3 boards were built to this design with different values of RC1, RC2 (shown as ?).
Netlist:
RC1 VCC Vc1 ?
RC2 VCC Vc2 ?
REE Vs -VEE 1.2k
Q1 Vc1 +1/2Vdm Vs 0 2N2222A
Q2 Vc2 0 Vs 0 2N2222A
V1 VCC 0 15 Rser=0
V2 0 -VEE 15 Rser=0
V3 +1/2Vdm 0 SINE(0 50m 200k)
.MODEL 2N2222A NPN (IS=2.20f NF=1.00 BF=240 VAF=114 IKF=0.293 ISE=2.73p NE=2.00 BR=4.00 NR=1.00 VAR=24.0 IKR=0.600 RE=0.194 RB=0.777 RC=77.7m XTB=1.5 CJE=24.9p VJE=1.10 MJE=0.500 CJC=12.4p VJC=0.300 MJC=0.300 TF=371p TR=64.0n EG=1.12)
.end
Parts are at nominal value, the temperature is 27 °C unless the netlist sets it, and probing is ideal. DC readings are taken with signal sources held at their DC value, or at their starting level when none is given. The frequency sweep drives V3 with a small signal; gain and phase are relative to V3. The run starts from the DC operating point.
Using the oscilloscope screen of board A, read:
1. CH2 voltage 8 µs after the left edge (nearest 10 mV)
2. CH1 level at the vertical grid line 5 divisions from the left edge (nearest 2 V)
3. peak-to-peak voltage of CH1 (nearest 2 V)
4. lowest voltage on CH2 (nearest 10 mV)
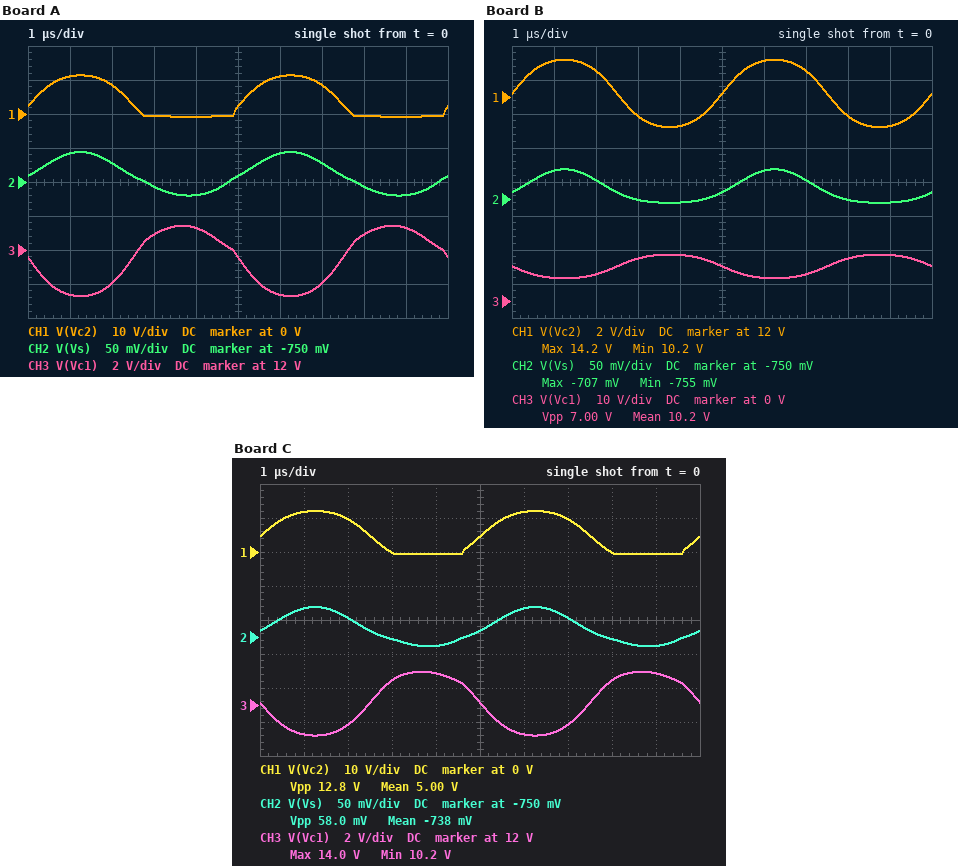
-760 mV
2 V
12 V
-770 mV
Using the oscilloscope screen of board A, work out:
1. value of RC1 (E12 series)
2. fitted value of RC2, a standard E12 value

560 Ω
2.2 kΩ
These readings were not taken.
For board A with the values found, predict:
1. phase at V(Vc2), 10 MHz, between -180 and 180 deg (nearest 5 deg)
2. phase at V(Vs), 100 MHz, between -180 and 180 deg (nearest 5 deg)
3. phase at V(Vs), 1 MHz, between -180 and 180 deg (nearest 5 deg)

-45 deg
0 deg
0 deg
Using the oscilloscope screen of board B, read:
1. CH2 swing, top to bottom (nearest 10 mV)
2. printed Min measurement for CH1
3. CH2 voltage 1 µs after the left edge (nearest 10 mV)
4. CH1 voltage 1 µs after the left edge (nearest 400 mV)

50 mV
10.2 V
-710 mV
14.0 V
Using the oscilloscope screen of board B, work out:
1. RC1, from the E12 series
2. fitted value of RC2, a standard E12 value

820 Ω
470 Ω
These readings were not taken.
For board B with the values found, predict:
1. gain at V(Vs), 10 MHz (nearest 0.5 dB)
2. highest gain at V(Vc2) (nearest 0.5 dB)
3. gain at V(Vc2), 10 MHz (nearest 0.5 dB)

-6.0 dB
34.0 dB
33.5 dB
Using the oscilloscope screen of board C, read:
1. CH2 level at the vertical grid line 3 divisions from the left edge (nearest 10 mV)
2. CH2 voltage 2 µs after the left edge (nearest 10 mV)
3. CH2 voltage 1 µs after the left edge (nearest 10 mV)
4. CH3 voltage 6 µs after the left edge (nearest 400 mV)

-750 mV
-720 mV
-710 mV
10.4 V
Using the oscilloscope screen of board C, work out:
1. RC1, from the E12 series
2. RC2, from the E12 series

470 Ω
1.8 kΩ
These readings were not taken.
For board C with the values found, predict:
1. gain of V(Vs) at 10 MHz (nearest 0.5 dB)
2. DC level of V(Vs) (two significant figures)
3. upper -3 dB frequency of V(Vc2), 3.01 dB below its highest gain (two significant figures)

-5.5 dB
-740 mV
16 MHz
